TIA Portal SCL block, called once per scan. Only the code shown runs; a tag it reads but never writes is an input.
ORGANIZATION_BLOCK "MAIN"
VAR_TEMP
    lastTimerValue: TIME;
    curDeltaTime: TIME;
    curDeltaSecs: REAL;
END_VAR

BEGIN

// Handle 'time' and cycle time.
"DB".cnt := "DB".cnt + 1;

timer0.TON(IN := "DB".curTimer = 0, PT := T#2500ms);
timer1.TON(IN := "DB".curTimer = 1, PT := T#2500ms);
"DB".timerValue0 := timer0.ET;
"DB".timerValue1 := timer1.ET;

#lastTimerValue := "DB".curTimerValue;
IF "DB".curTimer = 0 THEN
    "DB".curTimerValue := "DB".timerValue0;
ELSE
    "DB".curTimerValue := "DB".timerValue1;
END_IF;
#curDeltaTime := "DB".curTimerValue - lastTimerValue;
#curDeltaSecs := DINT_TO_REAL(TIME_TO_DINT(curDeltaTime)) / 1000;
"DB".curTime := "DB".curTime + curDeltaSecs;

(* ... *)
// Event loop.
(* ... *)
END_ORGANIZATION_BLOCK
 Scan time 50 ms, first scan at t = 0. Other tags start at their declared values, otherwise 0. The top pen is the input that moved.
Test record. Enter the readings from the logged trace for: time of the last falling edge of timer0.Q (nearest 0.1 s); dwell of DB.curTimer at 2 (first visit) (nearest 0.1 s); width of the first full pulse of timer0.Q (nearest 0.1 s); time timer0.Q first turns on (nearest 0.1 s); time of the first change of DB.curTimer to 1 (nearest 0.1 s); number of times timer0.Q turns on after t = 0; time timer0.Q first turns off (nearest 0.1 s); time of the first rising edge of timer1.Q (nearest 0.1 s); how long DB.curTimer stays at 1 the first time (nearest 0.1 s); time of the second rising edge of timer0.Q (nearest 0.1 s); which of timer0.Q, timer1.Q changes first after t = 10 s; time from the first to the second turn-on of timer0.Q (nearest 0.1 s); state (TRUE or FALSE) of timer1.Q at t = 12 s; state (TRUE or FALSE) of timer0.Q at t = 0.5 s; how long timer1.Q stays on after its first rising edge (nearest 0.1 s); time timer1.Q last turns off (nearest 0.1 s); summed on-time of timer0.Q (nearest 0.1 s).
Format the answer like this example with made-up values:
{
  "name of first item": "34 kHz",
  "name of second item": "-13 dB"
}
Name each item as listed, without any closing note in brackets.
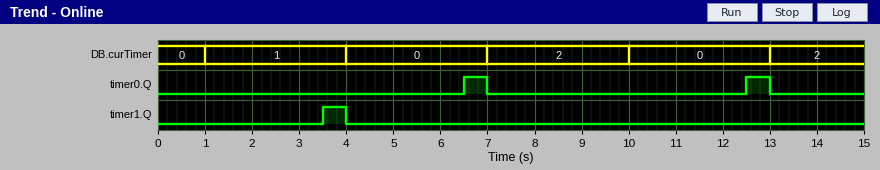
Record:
{
  "time of the last falling edge of timer0.Q": "13.0 s",
  "dwell of DB.curTimer at 2 (first visit)": "3.0 s",
  "width of the first full pulse of timer0.Q": "0.5 s",
  "time timer0.Q first turns on": "6.5 s",
  "time of the first change of DB.curTimer to 1": "1.0 s",
  "number of times timer0.Q turns on after t = 0": "2",
  "time timer0.Q first turns off": "7.0 s",
  "time of the first rising edge of timer1.Q": "3.5 s",
  "how long DB.curTimer stays at 1 the first time": "3.0 s",
  "time of the second rising edge of timer0.Q": "12.5 s",
  "which of timer0.Q, timer1.Q changes first after t = 10 s": "timer0.Q",
  "time from the first to the second turn-on of timer0.Q": "6.0 s",
  "state (TRUE or FALSE) of timer1.Q at t = 12 s": "FALSE",
  "state (TRUE or FALSE) of timer0.Q at t = 0.5 s": "FALSE",
  "how long timer1.Q stays on after its first rising edge": "0.5 s",
  "time timer1.Q last turns off": "4.0 s",
  "summed on-time of timer0.Q": "1.0 s"
}
